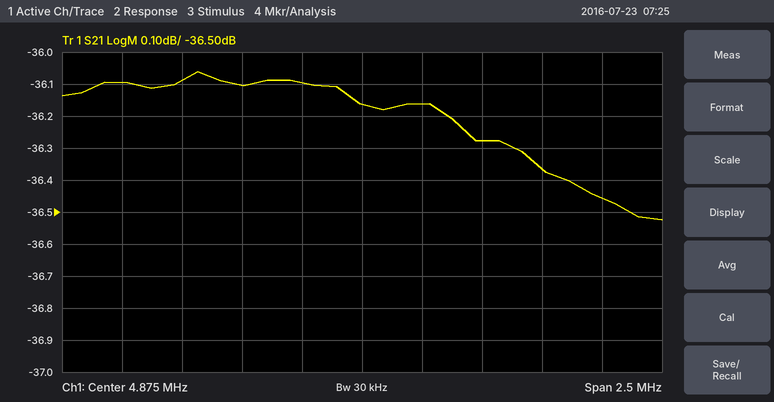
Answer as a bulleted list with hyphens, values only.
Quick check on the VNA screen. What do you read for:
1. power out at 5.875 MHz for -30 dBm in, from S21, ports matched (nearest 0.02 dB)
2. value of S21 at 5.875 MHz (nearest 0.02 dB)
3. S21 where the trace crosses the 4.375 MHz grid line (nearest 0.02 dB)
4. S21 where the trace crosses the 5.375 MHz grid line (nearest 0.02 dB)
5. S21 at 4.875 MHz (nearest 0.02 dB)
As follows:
- -66.46 dBm
- -36.46 dB
- -36.10 dB
- -36.28 dB
- -36.16 dB
